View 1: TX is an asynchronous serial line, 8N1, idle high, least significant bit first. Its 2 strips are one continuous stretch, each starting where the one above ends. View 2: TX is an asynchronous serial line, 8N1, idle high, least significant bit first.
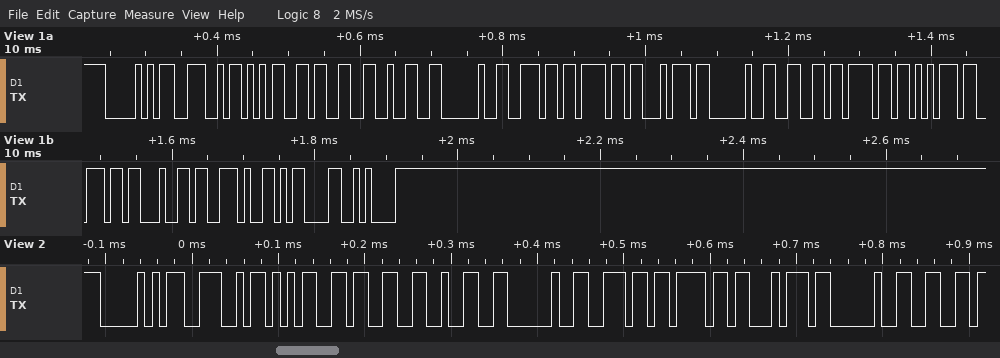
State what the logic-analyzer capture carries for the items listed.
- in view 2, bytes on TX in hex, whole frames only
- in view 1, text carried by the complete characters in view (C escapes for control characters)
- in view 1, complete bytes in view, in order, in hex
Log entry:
0x50 0x4E 0x35 0x33 0x32 0x20 0x6E 0x6F 0x74 0x20 0x66
"PN532 not found.\r\n"
0x50 0x4E 0x35 0x33 0x32 0x20 0x6E 0x6F 0x74 0x20 0x66 0x6F 0x75 0x6E 0x64 0x2E 0x0D 0x0A
